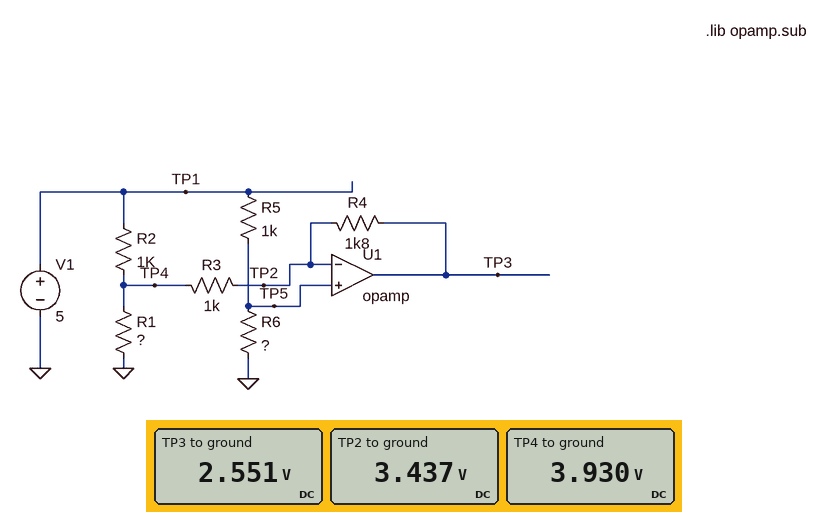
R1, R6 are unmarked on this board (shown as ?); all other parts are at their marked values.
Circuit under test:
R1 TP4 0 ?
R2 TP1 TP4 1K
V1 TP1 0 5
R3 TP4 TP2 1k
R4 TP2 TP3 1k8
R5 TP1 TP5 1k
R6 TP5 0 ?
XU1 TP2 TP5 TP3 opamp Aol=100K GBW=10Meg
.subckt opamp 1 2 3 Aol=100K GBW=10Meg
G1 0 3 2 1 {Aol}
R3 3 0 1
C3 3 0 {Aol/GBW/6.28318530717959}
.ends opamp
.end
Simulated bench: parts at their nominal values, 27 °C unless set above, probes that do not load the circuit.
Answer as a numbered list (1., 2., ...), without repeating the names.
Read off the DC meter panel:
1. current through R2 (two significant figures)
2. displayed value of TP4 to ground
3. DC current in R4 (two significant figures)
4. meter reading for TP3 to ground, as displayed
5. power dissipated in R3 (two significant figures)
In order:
1. 1.1 mA
2. 3.930 V
3. 490 µA
4. 2.551 V
5. 240 µW
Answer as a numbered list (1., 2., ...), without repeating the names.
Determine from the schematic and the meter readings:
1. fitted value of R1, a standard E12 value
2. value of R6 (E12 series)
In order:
1. 6.8 kΩ
2. 2.2 kΩ
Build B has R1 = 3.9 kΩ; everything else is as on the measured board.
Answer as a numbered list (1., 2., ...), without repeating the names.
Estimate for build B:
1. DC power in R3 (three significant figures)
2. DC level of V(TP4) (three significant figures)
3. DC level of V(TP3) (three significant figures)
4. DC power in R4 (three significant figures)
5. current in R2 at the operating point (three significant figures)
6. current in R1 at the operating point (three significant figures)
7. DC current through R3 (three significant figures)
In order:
1. 91.1 µW
2. 3.74 V
3. 2.89 V
4. 164 µW
5. 1.26 mA
6. 959 µA
7. 302 µA
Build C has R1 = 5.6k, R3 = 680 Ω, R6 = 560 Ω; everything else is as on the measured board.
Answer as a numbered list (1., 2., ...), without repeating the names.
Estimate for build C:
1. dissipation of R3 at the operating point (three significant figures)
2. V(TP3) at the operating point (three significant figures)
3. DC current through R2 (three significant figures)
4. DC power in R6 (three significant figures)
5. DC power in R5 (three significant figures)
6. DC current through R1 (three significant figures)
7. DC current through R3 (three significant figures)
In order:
1. 1.74 mW
2. -1.09 V
3. 2.12 mA
4. 5.75 mW
5. 10.3 mW
6. 515 µA
7. 1.60 mA
